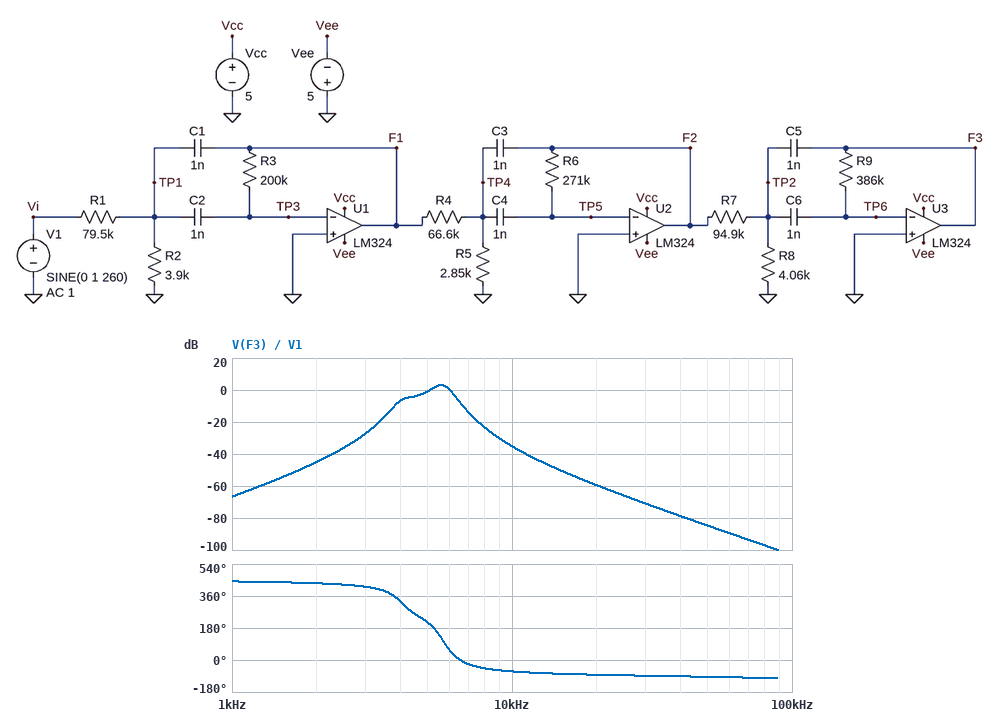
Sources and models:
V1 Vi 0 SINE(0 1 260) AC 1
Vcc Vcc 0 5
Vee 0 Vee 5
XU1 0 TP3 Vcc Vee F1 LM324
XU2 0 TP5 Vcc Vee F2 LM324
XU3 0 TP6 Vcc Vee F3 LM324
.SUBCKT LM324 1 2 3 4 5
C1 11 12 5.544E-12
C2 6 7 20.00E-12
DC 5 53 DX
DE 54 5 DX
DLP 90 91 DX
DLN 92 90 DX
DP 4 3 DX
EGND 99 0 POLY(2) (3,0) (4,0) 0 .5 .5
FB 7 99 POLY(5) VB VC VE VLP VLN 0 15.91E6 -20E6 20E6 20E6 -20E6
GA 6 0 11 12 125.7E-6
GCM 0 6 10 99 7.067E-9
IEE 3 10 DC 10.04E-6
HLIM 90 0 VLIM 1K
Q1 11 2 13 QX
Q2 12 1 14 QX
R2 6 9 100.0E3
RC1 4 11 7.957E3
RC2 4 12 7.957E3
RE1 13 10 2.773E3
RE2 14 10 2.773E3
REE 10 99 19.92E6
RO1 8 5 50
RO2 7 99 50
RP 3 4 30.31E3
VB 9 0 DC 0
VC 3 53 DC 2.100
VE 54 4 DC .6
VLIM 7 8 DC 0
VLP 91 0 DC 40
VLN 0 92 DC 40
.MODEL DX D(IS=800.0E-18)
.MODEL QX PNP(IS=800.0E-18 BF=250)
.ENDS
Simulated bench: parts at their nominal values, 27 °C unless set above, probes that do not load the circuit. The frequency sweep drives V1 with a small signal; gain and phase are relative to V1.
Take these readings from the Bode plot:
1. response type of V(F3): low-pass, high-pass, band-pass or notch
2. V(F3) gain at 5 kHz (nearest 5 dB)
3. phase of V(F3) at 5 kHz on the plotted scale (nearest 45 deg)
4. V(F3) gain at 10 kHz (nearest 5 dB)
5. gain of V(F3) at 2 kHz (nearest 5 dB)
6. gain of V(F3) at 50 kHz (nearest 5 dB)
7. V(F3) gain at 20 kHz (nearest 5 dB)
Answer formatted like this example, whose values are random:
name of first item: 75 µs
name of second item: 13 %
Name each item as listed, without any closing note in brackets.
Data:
response type of V(F3): low-pass, high-pass, band-pass or notch: band-pass
V(F3) gain at 5 kHz: 0 dB
phase of V(F3) at 5 kHz on the plotted scale: 225 deg
V(F3) gain at 10 kHz: -35 dB
gain of V(F3) at 2 kHz: -45 dB
gain of V(F3) at 50 kHz: -85 dB
V(F3) gain at 20 kHz: -60 dB
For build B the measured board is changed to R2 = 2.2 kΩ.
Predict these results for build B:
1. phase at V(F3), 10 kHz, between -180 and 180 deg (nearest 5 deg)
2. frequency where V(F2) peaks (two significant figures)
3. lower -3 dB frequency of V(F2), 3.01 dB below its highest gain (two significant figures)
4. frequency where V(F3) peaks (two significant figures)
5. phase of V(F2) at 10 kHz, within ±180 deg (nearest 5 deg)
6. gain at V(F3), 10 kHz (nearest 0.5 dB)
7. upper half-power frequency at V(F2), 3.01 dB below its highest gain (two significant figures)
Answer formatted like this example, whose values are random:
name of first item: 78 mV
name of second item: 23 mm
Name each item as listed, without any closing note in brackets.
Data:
phase at V(F3), 10 kHz, between -180 and 180 deg: -60 deg
frequency where V(F2) peaks: 5.9 kHz
lower -3 dB frequency of V(F2), 3.01 dB below its highest gain: 5.4 kHz
frequency where V(F3) peaks: 5.7 kHz
phase of V(F2) at 10 kHz, within ±180 deg: -155 deg
gain at V(F3), 10 kHz: -32.0 dB
upper half-power frequency at V(F2), 3.01 dB below its highest gain: 7.8 kHz
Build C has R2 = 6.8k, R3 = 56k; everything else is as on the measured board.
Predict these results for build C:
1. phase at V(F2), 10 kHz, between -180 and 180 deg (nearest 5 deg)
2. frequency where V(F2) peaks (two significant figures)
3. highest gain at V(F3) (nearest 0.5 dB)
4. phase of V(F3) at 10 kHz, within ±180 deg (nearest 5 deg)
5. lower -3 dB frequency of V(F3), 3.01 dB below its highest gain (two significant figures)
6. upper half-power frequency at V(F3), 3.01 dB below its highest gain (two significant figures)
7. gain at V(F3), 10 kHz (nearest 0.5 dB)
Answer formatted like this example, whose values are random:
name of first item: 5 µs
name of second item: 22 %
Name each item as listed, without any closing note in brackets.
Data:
phase at V(F2), 10 kHz, between -180 and 180 deg: -110 deg
frequency where V(F2) peaks: 5.8 kHz
highest gain at V(F3): -12.0 dB
phase of V(F3) at 10 kHz, within ±180 deg: -15 deg
lower -3 dB frequency of V(F3), 3.01 dB below its highest gain: 4.9 kHz
upper half-power frequency at V(F3), 3.01 dB below its highest gain: 6.2 kHz
gain at V(F3), 10 kHz: -34.0 dB
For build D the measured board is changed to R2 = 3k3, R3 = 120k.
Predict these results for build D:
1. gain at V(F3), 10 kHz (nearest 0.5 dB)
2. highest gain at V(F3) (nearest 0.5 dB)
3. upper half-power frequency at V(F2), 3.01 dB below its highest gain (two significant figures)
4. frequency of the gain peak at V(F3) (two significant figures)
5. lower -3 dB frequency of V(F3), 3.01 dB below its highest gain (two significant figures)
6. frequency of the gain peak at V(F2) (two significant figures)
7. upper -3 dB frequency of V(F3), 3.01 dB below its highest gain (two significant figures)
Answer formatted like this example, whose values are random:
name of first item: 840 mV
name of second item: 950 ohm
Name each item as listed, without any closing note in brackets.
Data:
gain at V(F3), 10 kHz: -31.5 dB
highest gain at V(F3): -9.0 dB
upper half-power frequency at V(F2), 3.01 dB below its highest gain: 7.5 kHz
frequency of the gain peak at V(F3): 5.7 kHz
lower -3 dB frequency of V(F3), 3.01 dB below its highest gain: 5.0 kHz
frequency of the gain peak at V(F2): 5.8 kHz
upper -3 dB frequency of V(F3), 3.01 dB below its highest gain: 6.3 kHz
